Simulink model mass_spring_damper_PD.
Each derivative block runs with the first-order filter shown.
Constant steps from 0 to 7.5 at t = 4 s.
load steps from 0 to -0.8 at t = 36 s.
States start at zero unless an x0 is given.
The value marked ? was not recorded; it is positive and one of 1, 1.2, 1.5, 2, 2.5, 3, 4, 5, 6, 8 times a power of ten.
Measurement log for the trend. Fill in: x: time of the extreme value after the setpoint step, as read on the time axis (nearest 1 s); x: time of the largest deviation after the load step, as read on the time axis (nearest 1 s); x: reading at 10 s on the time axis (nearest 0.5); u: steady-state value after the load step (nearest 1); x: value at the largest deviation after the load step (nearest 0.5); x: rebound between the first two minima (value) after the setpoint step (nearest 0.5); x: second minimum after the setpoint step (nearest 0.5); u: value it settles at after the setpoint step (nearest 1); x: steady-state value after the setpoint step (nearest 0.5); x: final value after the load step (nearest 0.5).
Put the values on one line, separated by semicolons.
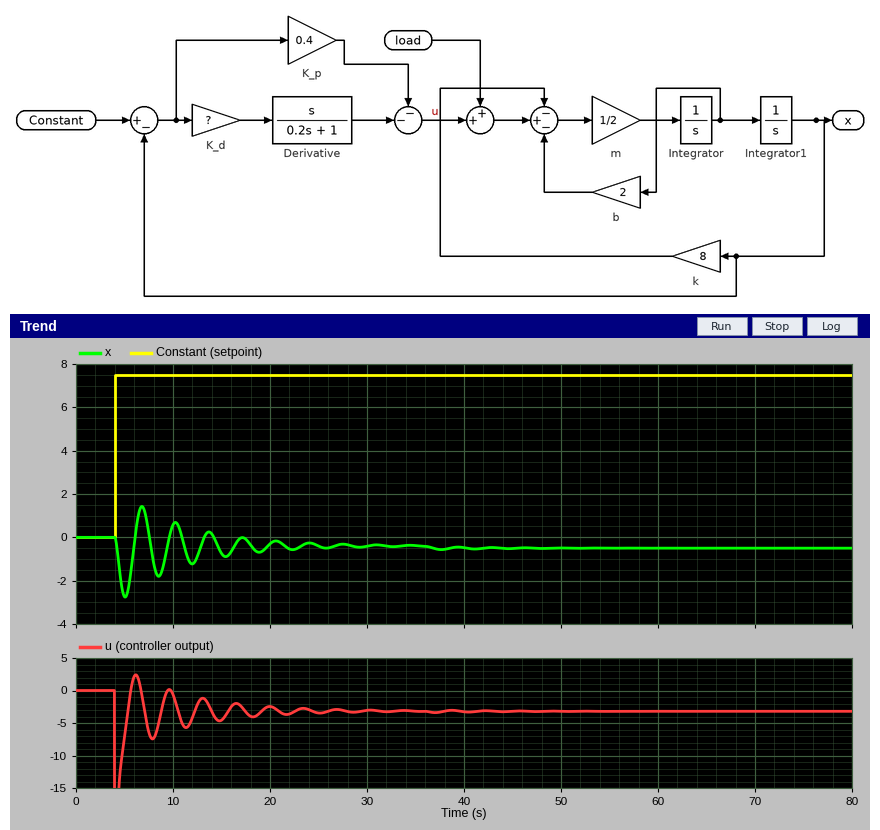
5 s; 38 s; 0.5; -3; -0.5; 1.5; -2.0; -3; -0.5; -0.5
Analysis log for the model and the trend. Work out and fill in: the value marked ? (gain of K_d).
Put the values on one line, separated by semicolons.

1.5
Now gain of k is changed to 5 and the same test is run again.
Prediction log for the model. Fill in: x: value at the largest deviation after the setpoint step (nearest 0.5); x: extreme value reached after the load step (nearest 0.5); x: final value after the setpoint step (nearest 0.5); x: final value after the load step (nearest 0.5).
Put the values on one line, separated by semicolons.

-3.5; -1.0; -0.5; -1.0
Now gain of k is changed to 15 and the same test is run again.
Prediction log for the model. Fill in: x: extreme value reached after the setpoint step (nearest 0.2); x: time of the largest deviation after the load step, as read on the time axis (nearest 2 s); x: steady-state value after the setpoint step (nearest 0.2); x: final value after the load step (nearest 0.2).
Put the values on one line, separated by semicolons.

-1.8; 38 s; -0.2; -0.2
